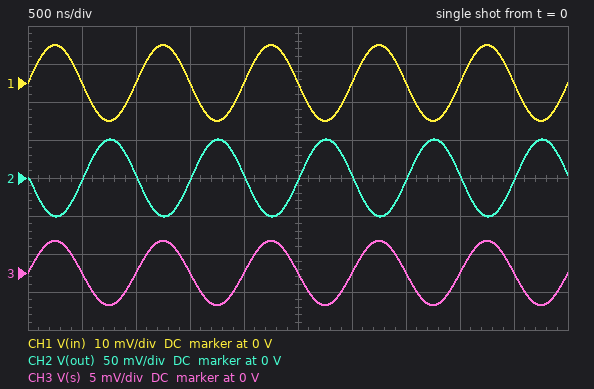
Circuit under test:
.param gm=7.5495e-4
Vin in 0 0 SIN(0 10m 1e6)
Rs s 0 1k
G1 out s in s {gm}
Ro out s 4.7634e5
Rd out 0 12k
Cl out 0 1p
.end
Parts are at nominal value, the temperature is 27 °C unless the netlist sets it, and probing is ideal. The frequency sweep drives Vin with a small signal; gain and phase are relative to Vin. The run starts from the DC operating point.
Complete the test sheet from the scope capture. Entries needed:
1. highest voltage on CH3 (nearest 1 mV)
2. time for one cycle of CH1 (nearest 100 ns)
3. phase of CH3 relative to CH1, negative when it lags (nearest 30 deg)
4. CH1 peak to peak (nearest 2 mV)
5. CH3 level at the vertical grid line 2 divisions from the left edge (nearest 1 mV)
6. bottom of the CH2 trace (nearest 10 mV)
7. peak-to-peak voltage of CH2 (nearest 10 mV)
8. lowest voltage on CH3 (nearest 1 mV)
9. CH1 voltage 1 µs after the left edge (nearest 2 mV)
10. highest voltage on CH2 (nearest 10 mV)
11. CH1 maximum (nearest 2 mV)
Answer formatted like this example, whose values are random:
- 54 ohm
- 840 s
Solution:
- 4 mV
- 1.0 µs
- 0 deg
- 20 mV
- 0 V
- -50 mV
- 100 mV
- -4 mV
- 0 V
- 50 mV
- 10 mV
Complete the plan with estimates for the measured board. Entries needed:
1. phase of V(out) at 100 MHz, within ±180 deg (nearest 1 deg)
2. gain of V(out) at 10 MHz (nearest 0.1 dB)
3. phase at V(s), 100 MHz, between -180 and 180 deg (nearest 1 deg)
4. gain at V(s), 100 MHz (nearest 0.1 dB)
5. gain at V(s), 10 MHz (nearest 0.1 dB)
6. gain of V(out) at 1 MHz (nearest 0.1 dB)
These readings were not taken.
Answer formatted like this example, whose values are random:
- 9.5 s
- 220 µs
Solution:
- 98 deg
- 12.2 dB
- 0 deg
- -7.3 dB
- -7.4 dB
- 14.1 dB
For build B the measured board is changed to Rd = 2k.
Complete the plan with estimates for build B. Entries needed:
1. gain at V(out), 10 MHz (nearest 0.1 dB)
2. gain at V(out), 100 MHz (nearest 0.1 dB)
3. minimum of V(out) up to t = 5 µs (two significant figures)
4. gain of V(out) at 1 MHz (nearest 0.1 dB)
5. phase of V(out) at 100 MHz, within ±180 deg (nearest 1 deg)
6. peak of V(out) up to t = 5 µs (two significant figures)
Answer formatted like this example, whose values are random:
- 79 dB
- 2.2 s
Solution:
- -1.4 dB
- -5.4 dB
- -8.6 mV
- -1.3 dB
- 129 deg
- 8.6 mV
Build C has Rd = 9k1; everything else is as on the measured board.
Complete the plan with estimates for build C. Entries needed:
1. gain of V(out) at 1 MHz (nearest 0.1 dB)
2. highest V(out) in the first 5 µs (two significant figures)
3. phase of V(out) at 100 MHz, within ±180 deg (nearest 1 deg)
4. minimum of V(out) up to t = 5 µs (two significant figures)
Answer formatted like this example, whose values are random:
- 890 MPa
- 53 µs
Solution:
- 11.7 dB
- 39 mV
- 100 deg
- -39 mV
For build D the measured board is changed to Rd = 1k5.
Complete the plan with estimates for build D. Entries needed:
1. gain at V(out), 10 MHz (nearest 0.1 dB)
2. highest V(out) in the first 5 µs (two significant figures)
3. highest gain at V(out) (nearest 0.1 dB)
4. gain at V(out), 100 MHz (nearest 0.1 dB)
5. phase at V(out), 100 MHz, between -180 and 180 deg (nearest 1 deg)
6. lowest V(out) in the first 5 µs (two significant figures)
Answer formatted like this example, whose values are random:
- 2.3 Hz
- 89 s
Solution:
- -3.9 dB
- 6.4 mV
- -3.8 dB
- -6.6 dB
- 137 deg
- -6.4 mV
